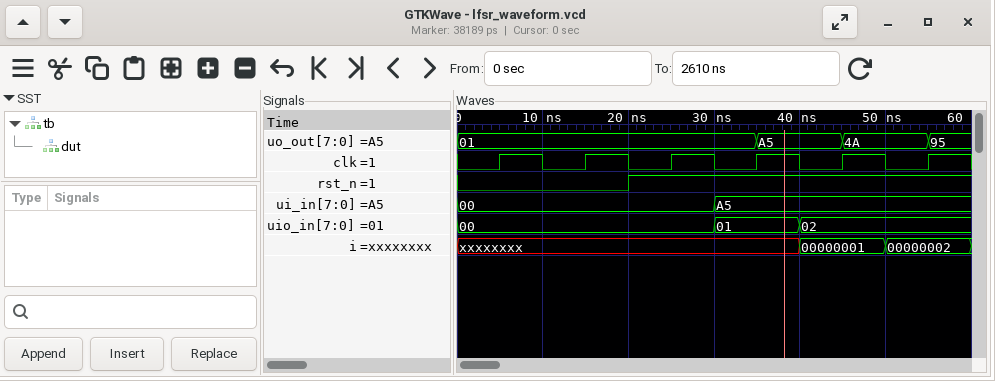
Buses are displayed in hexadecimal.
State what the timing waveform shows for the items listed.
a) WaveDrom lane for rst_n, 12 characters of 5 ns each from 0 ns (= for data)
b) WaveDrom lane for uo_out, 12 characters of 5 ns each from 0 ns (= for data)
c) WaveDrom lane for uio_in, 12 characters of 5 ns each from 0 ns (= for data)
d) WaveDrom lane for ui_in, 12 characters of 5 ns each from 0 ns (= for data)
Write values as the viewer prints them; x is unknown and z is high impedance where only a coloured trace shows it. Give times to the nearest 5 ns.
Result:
{name: 'rst_n', wave: '0...1.......'}
{name: 'uo_out', wave: '=......=.=.=', data: '01 A5 4A 95'}
{name: 'uio_in', wave: '=.....=.=...', data: '00 01 02'}
{name: 'ui_in', wave: '=.....=.....', data: '00 A5'}
